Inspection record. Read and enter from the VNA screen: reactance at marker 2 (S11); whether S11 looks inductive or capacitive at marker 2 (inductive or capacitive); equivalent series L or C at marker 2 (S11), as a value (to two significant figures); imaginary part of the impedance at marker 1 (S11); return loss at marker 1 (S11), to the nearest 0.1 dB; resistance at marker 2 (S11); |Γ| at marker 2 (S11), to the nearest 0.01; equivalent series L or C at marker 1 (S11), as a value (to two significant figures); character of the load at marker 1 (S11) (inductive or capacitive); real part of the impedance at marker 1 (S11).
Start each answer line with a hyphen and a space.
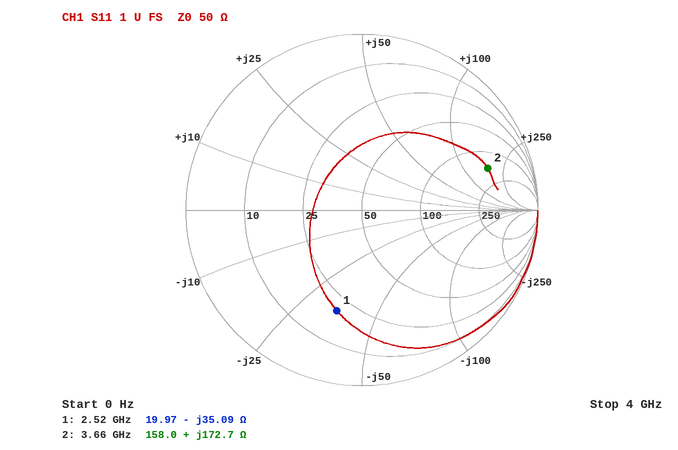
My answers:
- +172.7 Ω
- inductive
- 7.5 nH
- -35.09 Ω
- 4.6 dB
- 158.0 Ω
- 0.75
- 1.8 pF
- capacitive
- 19.97 Ω
